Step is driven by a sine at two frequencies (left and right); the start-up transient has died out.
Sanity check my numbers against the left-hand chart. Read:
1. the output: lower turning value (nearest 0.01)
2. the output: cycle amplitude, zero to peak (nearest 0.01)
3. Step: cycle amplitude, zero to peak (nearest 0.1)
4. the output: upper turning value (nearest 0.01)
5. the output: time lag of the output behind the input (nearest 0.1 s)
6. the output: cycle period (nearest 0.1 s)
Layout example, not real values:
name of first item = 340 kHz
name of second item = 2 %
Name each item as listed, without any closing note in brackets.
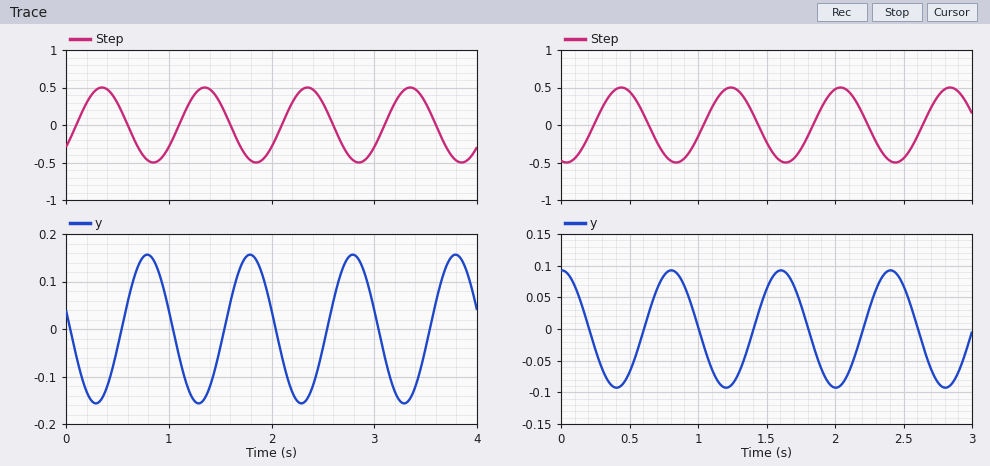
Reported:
the output: lower turning value = -0.16
the output: cycle amplitude, zero to peak = 0.16
Step: cycle amplitude, zero to peak = 0.5
the output: upper turning value = 0.16
the output: time lag of the output behind the input = 0.4 s
the output: cycle period = 1.0 s
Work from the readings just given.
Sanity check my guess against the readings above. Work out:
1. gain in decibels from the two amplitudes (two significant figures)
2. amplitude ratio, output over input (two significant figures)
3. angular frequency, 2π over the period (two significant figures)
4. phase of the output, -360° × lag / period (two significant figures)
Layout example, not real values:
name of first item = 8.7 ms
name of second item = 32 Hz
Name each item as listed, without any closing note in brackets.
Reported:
gain in decibels from the two amplitudes = -9.9 dB
amplitude ratio, output over input = 0.32
angular frequency, 2π over the period = 6.3 rad/s
phase of the output, -360° × lag / period = -140°
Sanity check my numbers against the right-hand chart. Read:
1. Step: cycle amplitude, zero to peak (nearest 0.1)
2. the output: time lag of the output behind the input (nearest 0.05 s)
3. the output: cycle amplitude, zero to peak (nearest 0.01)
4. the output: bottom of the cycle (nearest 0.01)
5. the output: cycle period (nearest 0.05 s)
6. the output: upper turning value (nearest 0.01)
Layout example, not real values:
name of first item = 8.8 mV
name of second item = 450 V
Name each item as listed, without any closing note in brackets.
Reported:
Step: cycle amplitude, zero to peak = 0.5
the output: time lag of the output behind the input = 0.35 s
the output: cycle amplitude, zero to peak = 0.09
the output: bottom of the cycle = -0.09
the output: cycle period = 0.80 s
the output: upper turning value = 0.09
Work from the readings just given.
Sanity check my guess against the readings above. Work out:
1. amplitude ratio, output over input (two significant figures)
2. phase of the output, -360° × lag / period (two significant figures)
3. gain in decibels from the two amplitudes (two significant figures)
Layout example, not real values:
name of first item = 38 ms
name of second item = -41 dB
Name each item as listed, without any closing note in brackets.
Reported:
amplitude ratio, output over input = 0.18
phase of the output, -360° × lag / period = -160°
gain in decibels from the two amplitudes = -15 dB
